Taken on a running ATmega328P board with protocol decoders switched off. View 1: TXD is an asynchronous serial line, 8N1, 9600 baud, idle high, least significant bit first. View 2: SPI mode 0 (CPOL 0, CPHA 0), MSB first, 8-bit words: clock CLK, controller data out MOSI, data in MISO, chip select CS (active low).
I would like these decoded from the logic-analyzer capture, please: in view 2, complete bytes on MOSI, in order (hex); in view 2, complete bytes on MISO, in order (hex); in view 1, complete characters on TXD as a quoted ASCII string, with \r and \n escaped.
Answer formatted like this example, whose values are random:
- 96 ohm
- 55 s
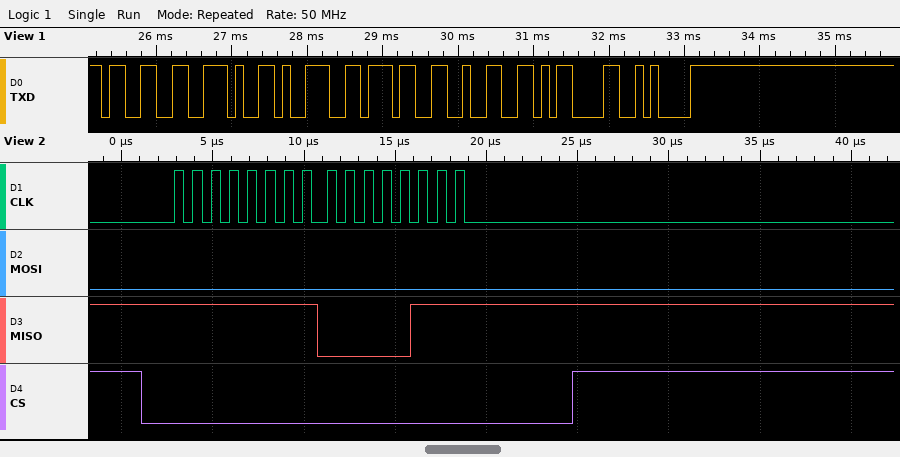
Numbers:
- 0x00 0x00
- 0xFF 0x07
- "3.972\r\n"
